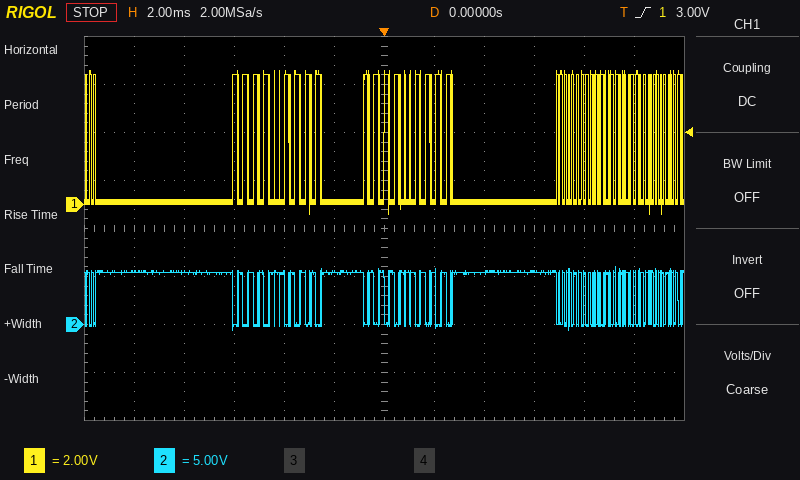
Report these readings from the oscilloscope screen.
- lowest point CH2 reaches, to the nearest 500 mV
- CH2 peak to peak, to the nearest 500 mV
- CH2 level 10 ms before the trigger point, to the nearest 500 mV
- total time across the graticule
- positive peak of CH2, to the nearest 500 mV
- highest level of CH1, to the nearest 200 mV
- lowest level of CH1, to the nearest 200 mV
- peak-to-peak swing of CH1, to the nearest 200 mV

-500 mV
6.5 V
5.5 V
24 ms
6.0 V
5.6 V
-400 mV
6.0 V
